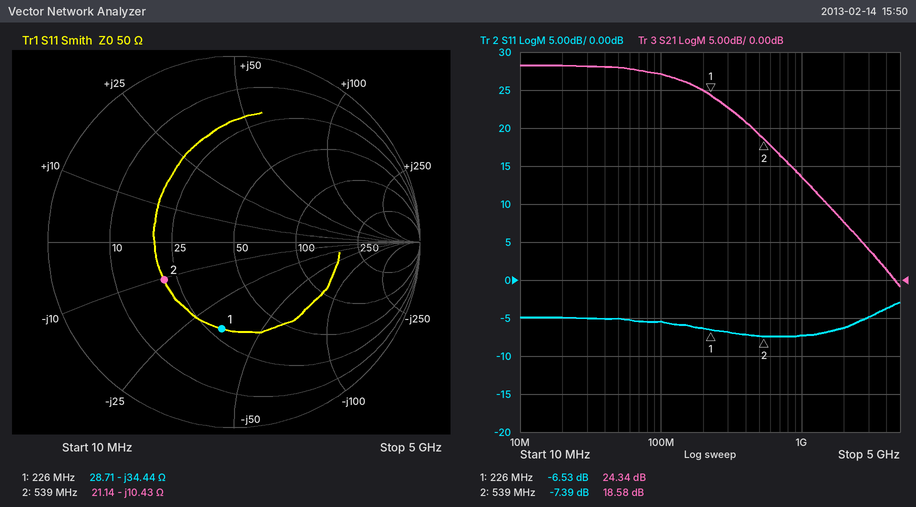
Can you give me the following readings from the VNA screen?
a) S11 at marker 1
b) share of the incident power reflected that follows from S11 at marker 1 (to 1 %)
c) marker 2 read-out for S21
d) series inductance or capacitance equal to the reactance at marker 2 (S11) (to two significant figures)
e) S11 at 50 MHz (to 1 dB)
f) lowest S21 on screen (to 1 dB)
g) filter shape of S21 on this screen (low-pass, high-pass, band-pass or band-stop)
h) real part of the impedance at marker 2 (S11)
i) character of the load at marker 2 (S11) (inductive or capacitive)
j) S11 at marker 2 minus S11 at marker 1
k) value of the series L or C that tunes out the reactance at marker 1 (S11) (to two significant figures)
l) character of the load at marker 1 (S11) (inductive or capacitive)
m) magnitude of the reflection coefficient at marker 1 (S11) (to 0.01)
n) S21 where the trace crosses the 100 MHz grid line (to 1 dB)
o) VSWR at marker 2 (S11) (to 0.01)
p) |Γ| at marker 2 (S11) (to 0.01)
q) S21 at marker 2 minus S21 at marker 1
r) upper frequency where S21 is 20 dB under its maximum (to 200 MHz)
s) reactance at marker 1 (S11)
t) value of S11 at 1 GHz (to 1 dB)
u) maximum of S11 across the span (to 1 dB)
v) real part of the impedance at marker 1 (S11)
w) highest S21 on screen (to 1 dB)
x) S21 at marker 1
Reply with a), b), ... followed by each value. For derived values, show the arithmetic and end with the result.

a) -6.53 dB
b) 10^(-6.53/10) ≈ 22 %
c) 18.58 dB
d) C = 1/(2π × 539 MHz × 10.43 Ω) ≈ 28 pF
e) -5 dB
f) -1 dB
g) low-pass
h) 21.14 Ω
i) capacitive
j) -7.39 − (-6.53) = -0.86 dB
k) L = 34.44 Ω/(2π × 226 MHz) ≈ 24 nH
l) capacitive
m) 0.47
n) 27 dB
o) (1 + 0.4271)/(1 − 0.4271) ≈ 2.49
p) 0.43
q) 18.58 − (24.34) = -5.76 dB
r) 1.8 GHz
s) -34.44 Ω
t) -7 dB
u) -3 dB
v) 28.71 Ω
w) 28 dB
x) 24.34 dB
